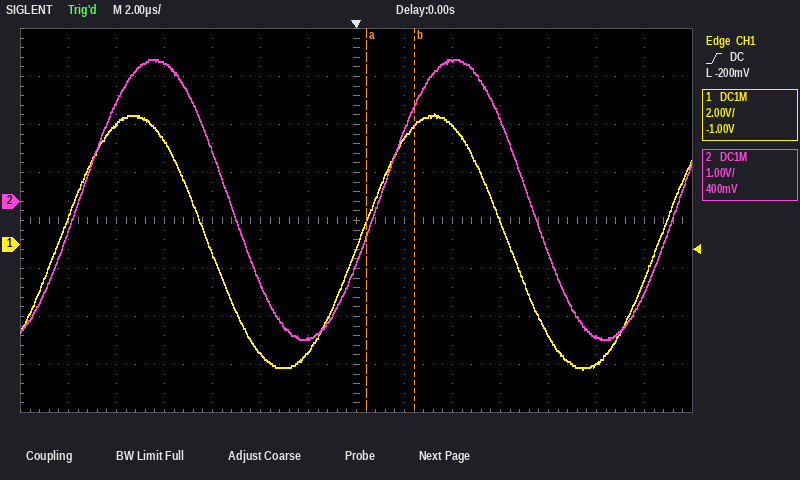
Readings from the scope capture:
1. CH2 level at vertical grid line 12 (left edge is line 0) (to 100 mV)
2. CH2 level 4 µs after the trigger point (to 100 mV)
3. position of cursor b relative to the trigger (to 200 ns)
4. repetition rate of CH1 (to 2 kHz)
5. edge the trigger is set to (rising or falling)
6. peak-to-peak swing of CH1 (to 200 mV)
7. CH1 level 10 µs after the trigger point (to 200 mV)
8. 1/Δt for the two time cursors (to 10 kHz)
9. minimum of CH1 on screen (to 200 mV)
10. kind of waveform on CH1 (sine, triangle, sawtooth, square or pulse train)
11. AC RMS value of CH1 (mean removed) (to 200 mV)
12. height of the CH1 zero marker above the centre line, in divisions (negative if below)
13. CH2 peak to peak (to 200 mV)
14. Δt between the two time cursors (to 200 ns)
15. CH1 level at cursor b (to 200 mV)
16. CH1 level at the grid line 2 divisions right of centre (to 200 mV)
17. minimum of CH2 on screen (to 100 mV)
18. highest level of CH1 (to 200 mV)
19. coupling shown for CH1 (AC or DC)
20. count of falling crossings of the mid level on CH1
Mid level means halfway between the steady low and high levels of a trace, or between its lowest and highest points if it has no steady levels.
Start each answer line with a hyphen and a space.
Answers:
- -2.8 V
- 2.9 V
- +2.4 µs
- 80 kHz
- rising
- 10.6 V
- -5.0 V
- 500 kHz
- -5.2 V
- sine
- 3.8 V
- -0.5 div
- 5.8 V
- 2.0 µs
- 5.0 V
- 5.0 V
- -2.9 V
- 5.4 V
- DC
- 2
